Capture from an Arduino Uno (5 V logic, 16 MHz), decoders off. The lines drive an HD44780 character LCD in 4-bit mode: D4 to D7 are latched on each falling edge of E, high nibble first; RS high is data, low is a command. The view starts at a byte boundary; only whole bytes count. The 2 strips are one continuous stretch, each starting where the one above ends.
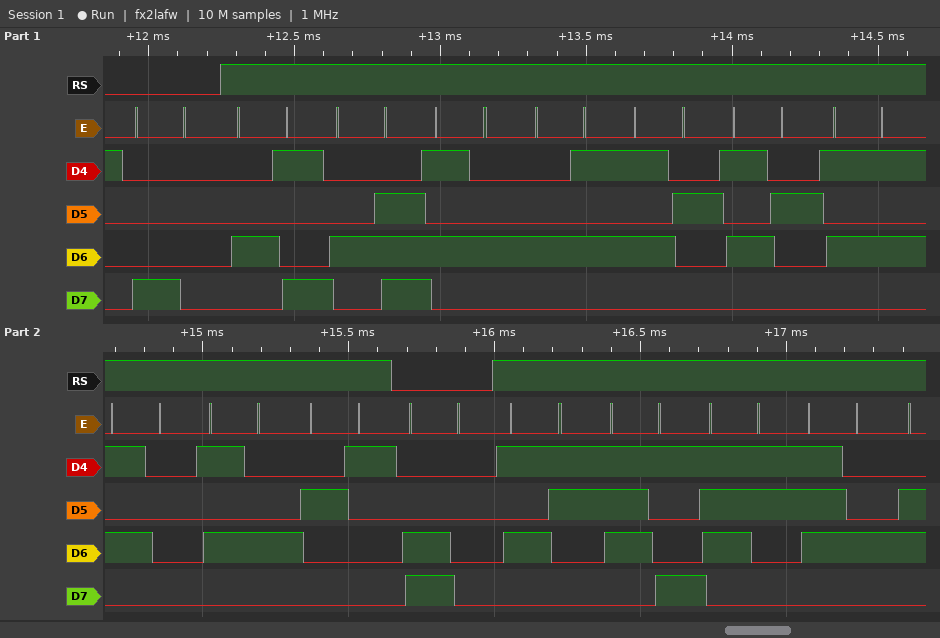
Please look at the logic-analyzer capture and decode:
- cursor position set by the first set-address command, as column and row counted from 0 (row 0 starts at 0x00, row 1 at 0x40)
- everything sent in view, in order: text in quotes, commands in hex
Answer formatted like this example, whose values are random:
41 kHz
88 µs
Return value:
column 0, row 0
0x80 "INTERRUPT!" 0xC0 "Syst"
